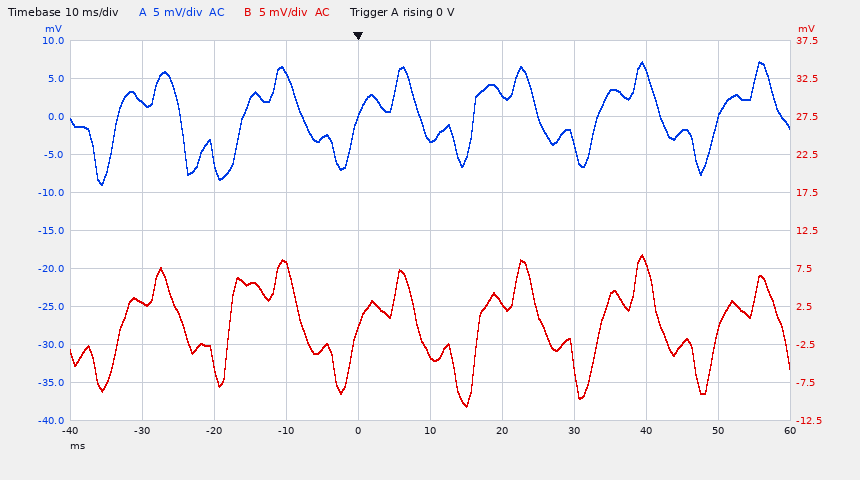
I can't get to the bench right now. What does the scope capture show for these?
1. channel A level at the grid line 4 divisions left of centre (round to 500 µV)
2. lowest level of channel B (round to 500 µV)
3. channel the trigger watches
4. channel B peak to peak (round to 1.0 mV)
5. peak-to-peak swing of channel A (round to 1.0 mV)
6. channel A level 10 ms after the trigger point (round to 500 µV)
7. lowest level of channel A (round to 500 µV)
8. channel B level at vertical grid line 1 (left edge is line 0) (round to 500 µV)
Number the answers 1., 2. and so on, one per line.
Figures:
1. 2.0 mV
2. -10.5 mV
3. channel A
4. 20.0 mV
5. 16.0 mV
6. -3.0 mV
7. -9.0 mV
8. 3.0 mV
